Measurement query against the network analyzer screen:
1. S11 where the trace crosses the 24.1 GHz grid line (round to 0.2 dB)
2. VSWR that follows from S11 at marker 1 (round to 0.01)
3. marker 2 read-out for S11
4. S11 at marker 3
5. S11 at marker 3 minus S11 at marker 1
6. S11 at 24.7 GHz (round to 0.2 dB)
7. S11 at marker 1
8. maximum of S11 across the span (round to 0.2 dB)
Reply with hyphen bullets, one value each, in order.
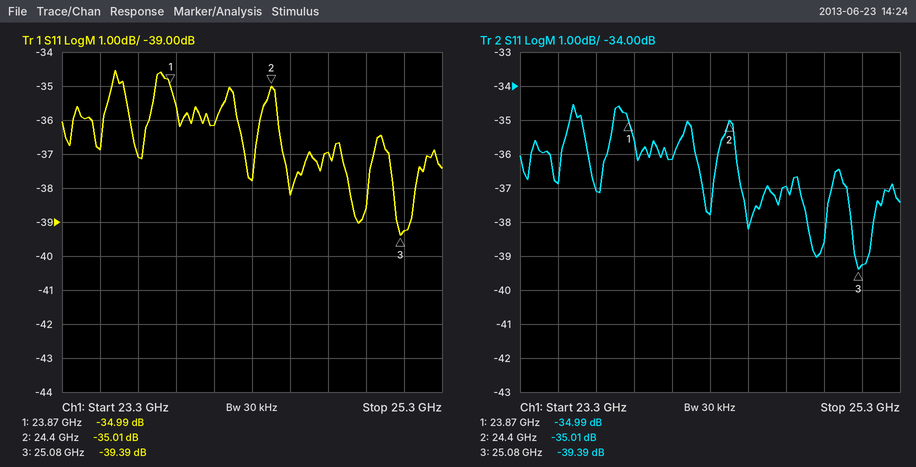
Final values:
- -36.2 dB
- 1.04
- -35.01 dB
- -39.39 dB
- -4.40 dB
- -37.0 dB
- -34.99 dB
- -34.6 dB
